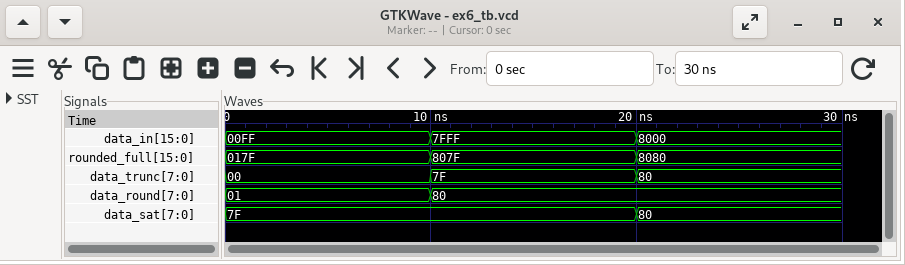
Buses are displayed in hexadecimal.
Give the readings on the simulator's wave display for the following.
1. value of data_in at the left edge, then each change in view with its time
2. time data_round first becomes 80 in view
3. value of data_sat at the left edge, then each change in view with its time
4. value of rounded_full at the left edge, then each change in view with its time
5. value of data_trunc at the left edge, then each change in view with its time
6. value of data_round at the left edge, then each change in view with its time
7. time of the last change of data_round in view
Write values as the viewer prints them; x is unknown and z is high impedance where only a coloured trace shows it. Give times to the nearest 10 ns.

00FF, 7FFF at 10 ns, 8000 at 20 ns
10 ns
7F, 80 at 20 ns
017F, 807F at 10 ns, 8080 at 20 ns
00, 7F at 10 ns, 80 at 20 ns
01, 80 at 10 ns
10 ns
